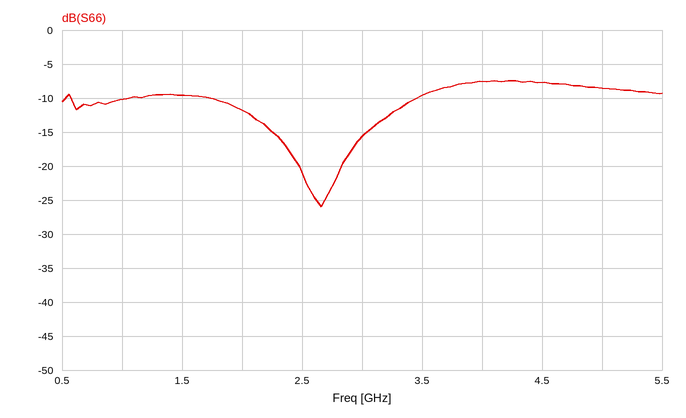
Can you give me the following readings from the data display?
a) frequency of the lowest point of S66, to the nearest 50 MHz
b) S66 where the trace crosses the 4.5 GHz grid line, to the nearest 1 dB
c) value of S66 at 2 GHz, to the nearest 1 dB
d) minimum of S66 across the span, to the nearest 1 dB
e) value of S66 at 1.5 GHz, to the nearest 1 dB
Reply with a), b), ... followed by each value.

a) 2.65 GHz
b) -8 dB
c) -12 dB
d) -26 dB
e) -10 dB
